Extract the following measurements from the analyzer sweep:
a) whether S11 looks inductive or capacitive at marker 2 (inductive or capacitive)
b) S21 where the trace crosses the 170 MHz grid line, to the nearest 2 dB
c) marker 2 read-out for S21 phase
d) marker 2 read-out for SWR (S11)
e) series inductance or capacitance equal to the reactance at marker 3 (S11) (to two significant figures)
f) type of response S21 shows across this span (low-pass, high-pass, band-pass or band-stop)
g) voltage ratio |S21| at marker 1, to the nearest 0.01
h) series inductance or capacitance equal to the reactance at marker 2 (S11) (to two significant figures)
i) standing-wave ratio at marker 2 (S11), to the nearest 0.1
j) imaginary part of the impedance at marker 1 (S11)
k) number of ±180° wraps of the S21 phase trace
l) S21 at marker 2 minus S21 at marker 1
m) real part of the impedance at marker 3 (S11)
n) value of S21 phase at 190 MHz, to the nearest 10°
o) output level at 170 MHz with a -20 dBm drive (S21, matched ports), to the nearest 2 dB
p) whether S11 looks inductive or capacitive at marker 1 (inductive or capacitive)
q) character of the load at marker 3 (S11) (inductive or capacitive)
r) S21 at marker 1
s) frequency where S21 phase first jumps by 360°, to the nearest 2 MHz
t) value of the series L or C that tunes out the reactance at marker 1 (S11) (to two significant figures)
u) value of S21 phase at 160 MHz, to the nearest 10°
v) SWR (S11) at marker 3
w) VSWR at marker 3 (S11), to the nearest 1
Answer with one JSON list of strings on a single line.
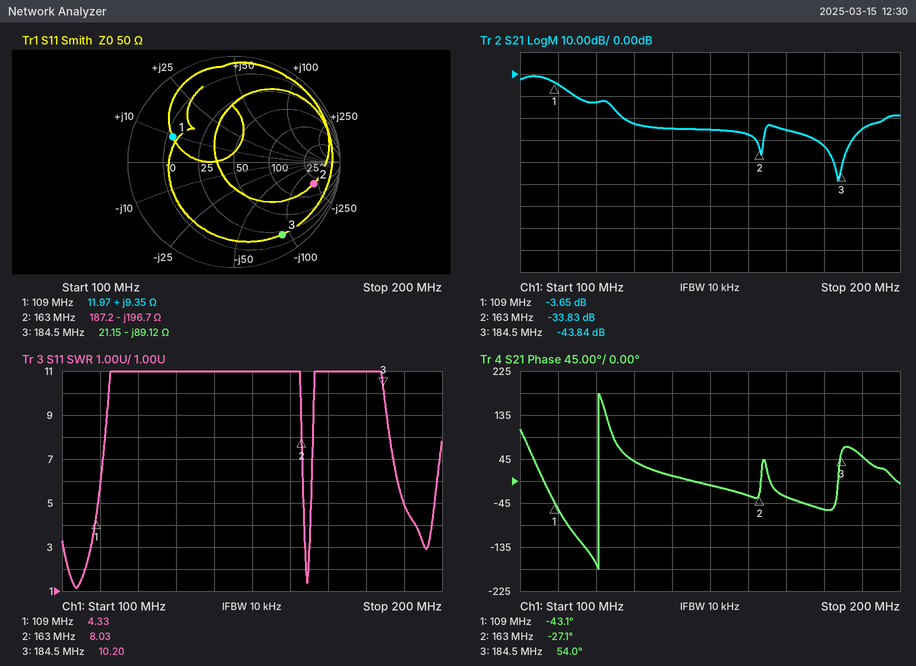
["capacitive", "-26 dB", "-27.1°", "8.03", "9.7 pF", "low-pass", "0.66", "5.0 pF", "8.0", "+9.35 Ω", "1", "-30.18 dB", "21.15 Ω", "50°", "-46 dBm", "inductive", "capacitive", "-3.65 dB", "120 MHz", "160 pF", "-30°", "10.20", "10"]
